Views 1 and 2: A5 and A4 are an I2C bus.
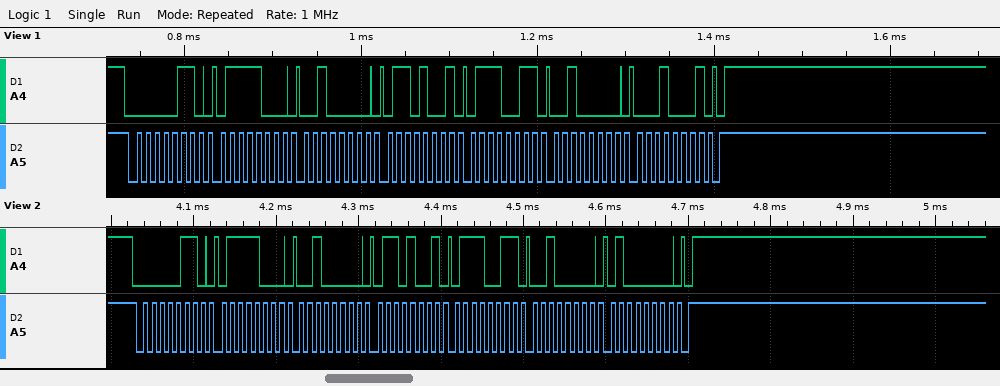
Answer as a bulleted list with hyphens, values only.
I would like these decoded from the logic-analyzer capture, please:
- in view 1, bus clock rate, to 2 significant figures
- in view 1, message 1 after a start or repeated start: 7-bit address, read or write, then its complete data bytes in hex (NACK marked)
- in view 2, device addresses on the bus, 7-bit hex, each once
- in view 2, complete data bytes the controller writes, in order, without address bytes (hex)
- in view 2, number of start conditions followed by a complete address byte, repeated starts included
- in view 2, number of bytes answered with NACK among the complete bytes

- 100 kHz
- 0x03 write: 78 20 69 73 20 11
- 0x03
- 78 20 69 73 20 40
- 1
- 0
